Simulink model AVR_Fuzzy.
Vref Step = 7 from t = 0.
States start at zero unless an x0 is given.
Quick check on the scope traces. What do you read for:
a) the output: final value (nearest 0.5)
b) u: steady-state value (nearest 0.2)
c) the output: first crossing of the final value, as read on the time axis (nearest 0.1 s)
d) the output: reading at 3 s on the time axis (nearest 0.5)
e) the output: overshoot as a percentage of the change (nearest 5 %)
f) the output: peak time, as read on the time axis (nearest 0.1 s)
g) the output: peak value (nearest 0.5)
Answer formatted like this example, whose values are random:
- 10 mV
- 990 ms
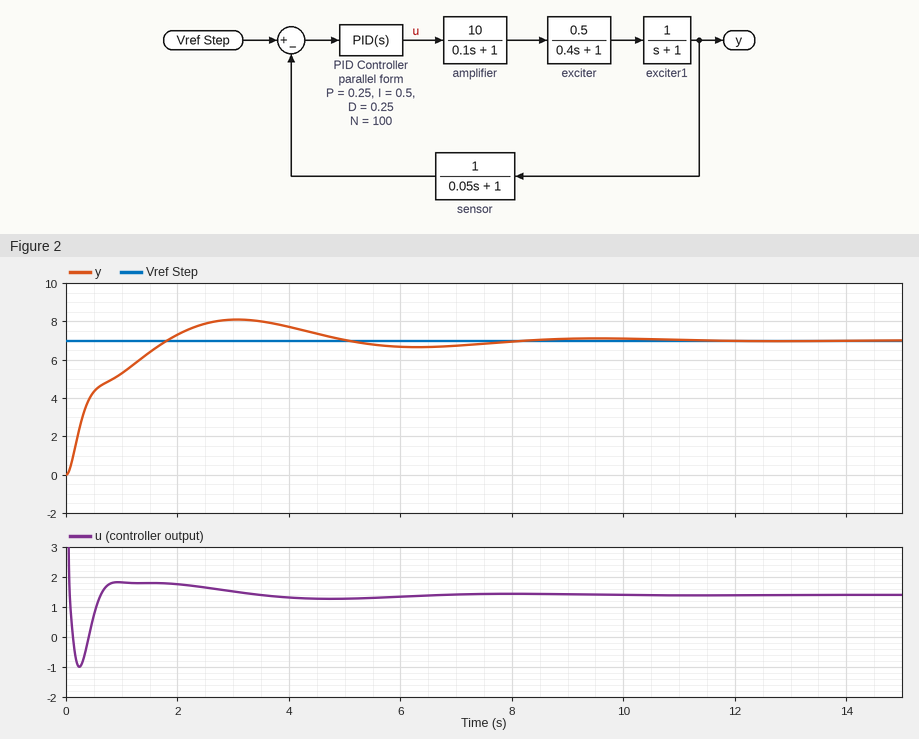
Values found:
- 7.0
- 1.4
- 1.8 s
- 8.0
- 15 %
- 3.1 s
- 8.0
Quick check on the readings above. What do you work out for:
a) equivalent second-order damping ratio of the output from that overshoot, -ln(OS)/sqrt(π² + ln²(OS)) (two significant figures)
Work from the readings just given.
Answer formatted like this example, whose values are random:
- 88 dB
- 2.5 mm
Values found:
- 0.52
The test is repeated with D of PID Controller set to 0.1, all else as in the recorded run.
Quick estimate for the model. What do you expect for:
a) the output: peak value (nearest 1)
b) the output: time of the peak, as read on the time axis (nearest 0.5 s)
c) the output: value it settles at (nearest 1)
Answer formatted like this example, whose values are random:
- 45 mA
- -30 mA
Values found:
- 9
- 2.5 s
- 7
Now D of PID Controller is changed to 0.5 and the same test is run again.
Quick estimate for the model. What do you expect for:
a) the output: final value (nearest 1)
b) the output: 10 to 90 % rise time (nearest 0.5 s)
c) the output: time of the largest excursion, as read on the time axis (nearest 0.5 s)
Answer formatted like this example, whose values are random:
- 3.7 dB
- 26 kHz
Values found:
- 7
- 2.0 s
- 4.0 s
